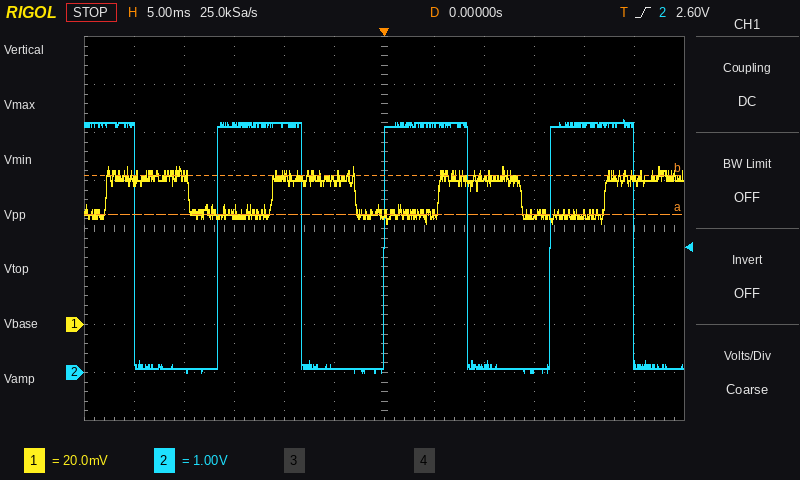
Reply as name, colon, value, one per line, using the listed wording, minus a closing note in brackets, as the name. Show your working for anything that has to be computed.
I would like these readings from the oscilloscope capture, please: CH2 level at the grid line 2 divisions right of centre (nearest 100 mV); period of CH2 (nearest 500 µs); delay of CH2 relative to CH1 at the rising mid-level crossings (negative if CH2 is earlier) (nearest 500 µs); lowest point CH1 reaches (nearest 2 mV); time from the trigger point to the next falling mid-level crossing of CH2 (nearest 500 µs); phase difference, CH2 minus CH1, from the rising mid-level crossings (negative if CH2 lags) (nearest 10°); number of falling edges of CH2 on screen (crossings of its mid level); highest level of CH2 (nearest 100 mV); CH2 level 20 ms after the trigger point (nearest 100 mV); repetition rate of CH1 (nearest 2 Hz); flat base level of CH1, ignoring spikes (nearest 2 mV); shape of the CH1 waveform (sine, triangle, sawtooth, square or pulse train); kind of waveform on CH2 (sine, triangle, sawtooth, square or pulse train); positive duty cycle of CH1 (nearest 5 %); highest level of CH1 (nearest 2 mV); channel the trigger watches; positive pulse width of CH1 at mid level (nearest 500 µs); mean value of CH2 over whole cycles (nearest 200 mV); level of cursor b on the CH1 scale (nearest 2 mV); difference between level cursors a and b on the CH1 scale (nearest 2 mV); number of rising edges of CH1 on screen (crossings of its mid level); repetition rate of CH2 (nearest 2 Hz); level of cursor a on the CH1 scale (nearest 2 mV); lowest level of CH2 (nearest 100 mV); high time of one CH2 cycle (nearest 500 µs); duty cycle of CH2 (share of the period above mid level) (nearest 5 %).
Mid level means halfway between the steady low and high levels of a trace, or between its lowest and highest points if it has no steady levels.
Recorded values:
CH2 level at the grid line 2 divisions right of centre: 100 mV
period of CH2: 16.5 ms
delay of CH2 relative to CH1 at the rising mid-level crossings (negative if CH2 is earlier): -5.5 ms
lowest point CH1 reaches: 42 mV
time from the trigger point to the next falling mid-level crossing of CH2: 8.5 ms
phase difference, CH2 minus CH1, from the rising mid-level crossings (negative if CH2 lags): −360° × (-5.5 ms) / 16.5 ms ≈ +120°
number of falling edges of CH2 on screen: 4
highest level of CH2: 5.3 V
CH2 level 20 ms after the trigger point: 5.2 V
repetition rate of CH1: 1 / 16.5 ms ≈ 60.6 Hz, so 60 Hz to the nearest 2 Hz
flat base level of CH1, ignoring spikes: 46 mV
shape of the CH1 waveform: square
kind of waveform on CH2: square
positive duty cycle of CH1: 8.5 ms / 16.5 ms ≈ 51.5 %, so 50 % to the nearest 5 %
highest level of CH1: 66 mV
channel the trigger watches: CH2
positive pulse width of CH1 at mid level: 8.5 ms
mean value of CH2 over whole cycles: 0.0 V + 0.5 × (5.3 V − (0.0 V)) ≈ 2.6 V
level of cursor b on the CH1 scale: 62 mV
difference between level cursors a and b on the CH1 scale: 16 mV
number of rising edges of CH1 on screen: 4
repetition rate of CH2: 1 / 16.5 ms ≈ 60.6 Hz, so 60 Hz to the nearest 2 Hz
level of cursor a on the CH1 scale: 46 mV
lowest level of CH2: 0.0 V
high time of one CH2 cycle: 8.5 ms
duty cycle of CH2 (share of the period above mid level): 8.5 ms / 16.5 ms ≈ 51.5 %, so 50 % to the nearest 5 %
